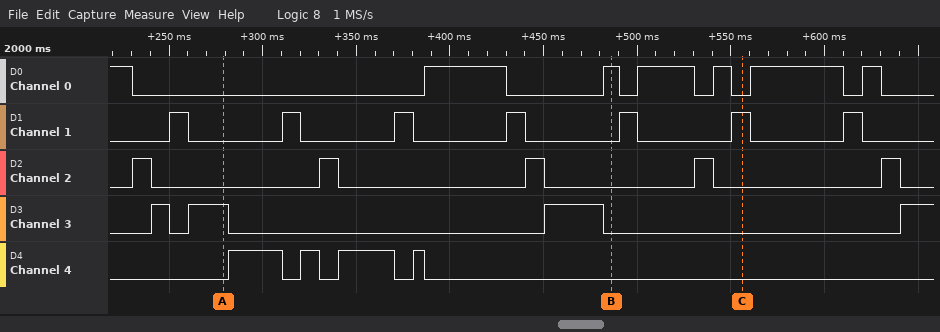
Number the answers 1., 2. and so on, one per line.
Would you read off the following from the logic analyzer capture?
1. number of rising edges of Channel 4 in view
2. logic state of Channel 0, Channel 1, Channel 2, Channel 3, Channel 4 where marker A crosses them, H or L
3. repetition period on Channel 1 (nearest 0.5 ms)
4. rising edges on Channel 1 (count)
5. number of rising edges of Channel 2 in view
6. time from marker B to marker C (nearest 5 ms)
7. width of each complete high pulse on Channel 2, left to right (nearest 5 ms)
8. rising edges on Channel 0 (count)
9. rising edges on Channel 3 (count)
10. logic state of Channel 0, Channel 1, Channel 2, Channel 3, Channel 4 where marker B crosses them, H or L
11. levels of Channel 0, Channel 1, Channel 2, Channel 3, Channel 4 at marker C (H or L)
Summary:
1. 4
2. Channel 0=L, Channel 1=L, Channel 2=L, Channel 3=H, Channel 4=L
3. 60 ms
4. 7
5. 5
6. 70 ms
7. 10 ms, 10 ms, 10 ms, 10 ms, 10 ms
8. 6
9. 4
10. Channel 0=H, Channel 1=L, Channel 2=L, Channel 3=L, Channel 4=L
11. Channel 0=L, Channel 1=H, Channel 2=L, Channel 3=L, Channel 4=L
